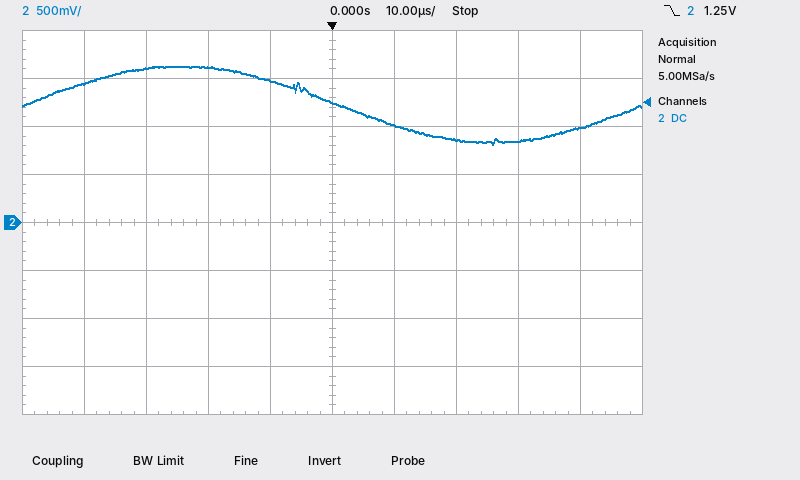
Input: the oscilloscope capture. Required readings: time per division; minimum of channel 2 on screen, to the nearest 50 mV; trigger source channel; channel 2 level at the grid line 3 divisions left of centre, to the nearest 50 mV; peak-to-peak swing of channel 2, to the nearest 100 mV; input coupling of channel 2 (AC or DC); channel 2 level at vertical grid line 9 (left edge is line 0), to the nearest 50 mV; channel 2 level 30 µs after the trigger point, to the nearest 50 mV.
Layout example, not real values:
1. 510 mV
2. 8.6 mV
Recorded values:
1. 10 µs
2. 800 mV
3. channel 2
4. 1.60 V
5. 800 mV
6. DC
7. 1.00 V
8. 850 mV
